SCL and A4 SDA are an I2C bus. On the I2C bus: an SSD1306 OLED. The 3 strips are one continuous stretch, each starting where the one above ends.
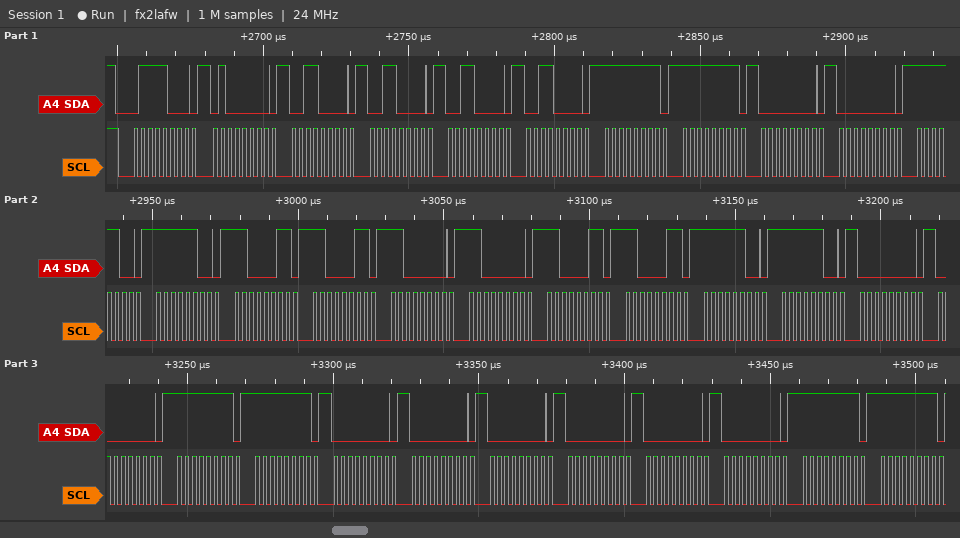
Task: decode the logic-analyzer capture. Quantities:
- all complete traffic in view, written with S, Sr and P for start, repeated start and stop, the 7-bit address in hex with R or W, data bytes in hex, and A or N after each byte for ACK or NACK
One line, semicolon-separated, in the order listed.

S 3CW A 40 A 30 A 30 A 30 A 30 A FF A FF A 00 A 00 A FC A FC A C3 A C3 A C0 A C0 A C3 A C3 A FC A FC A 00 A 00 A FF A FF A 00 A 00 A 00 A 00 A 00 A 00 A FF A FF A
